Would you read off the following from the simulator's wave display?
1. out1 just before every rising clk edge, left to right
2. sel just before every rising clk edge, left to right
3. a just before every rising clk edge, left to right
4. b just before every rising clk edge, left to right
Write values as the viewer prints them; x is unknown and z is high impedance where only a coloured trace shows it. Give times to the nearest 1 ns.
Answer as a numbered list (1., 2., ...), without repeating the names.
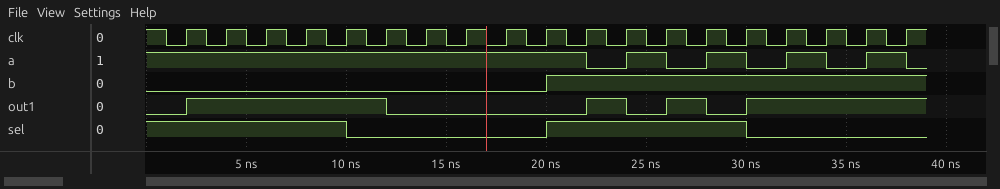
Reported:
1. 0 1 1 1 1 1 0 0 0 0 0 1 0 1 0 1 1 1 1
2. 1 1 1 1 1 0 0 0 0 0 1 1 1 1 1 0 0 0 0
3. 1 1 1 1 1 1 1 1 1 1 1 0 1 0 1 0 1 0 1
4. 0 0 0 0 0 0 0 0 0 0 1 1 1 1 1 1 1 1 1
